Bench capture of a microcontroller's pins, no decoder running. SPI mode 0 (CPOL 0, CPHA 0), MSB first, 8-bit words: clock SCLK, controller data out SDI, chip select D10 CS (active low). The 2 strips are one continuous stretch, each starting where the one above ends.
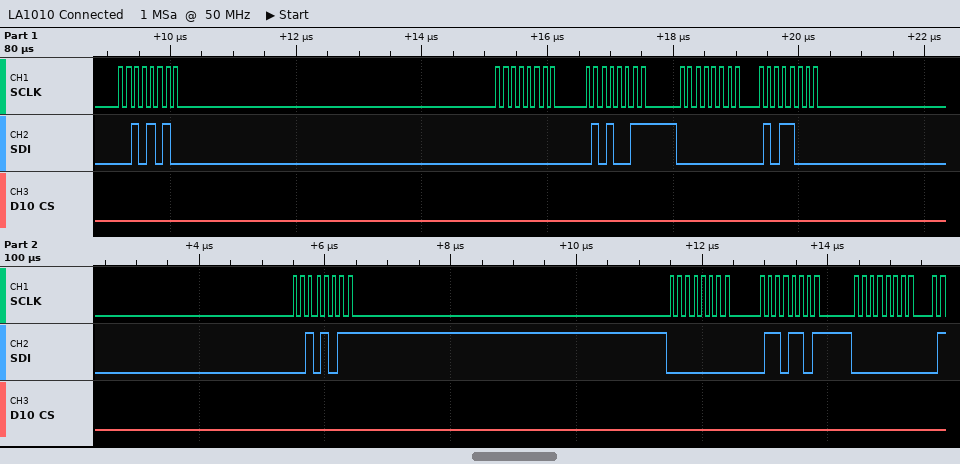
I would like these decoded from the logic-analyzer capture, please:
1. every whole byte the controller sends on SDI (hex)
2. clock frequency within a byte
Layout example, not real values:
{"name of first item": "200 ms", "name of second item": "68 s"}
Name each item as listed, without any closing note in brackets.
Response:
{"every whole byte the controller sends on SDI": "2A 00 53 00 58 2B 00 6D 00", "clock frequency within a byte": "8 MHz"}
